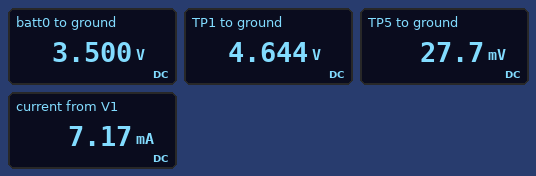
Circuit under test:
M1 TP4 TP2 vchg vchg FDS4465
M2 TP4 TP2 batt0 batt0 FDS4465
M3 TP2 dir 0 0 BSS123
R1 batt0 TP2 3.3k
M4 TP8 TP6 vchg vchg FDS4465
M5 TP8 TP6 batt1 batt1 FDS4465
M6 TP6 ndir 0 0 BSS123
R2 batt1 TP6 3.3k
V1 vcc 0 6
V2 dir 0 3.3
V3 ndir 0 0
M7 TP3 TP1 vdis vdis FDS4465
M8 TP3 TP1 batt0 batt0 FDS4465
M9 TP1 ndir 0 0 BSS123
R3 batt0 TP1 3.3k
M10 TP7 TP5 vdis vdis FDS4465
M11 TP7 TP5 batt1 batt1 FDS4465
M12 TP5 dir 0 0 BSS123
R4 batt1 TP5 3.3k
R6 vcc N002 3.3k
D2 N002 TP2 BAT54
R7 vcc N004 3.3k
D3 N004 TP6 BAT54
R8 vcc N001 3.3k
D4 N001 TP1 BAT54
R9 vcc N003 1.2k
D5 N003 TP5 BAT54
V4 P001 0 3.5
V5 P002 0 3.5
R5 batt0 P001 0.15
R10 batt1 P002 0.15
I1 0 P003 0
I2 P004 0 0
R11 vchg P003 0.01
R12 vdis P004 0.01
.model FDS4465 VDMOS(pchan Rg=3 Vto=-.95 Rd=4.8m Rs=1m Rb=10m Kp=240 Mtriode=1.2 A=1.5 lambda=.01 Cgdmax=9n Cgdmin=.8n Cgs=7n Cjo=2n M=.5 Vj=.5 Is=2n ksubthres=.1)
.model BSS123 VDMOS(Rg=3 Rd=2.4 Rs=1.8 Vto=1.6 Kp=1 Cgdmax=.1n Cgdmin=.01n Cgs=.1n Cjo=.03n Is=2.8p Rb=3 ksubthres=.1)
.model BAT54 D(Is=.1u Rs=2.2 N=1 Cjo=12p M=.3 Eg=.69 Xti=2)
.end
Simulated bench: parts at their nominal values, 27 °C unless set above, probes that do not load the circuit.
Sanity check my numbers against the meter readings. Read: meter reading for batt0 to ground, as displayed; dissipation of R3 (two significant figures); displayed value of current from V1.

3.500 V
400 µW
7.17 mA
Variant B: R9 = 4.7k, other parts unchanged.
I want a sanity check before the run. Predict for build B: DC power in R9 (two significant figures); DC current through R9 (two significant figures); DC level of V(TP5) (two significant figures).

7.0 mW
1.2 mA
11 mV
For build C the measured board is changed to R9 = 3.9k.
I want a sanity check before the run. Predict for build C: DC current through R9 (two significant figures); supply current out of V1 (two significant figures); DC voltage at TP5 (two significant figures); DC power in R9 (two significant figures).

1.5 mA
3.9 mA
12 mV
8.4 mW
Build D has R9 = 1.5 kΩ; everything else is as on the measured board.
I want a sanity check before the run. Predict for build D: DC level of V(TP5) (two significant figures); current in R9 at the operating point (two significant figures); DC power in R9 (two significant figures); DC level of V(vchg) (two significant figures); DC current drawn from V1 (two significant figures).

23 mV
3.8 mA
22 mW
3.5 V
6.2 mA
